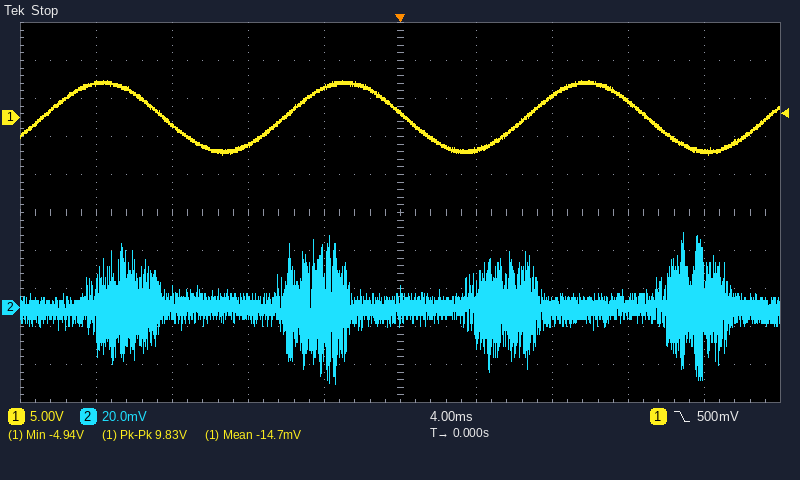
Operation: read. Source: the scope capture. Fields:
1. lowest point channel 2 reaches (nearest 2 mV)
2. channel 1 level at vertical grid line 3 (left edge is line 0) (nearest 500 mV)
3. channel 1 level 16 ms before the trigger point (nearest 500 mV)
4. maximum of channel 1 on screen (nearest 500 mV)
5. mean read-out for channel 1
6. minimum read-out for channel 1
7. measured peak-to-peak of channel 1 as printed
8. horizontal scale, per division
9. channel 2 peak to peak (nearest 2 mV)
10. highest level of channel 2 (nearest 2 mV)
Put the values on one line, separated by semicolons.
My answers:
-40 mV; -3.5 V; 4.5 V; 5.0 V; -14.7 mV; -4.94 V; 9.83 V; 4 ms; 80 mV; 40 mV
